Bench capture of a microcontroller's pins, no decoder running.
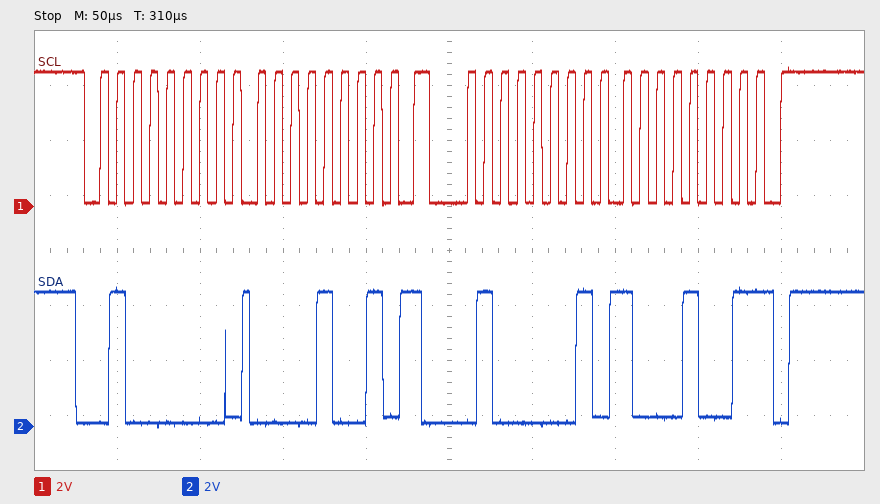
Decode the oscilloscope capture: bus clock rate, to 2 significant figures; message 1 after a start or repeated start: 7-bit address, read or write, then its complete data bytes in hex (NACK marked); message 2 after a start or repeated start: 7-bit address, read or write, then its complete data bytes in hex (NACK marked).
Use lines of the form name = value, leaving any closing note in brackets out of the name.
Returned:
bus clock rate, to 2 significant figures = 100 kHz
message 1 after a start or repeated start: 7-bit address, read or write, then its complete data bytes in hex = 0x20 write: 09
message 2 after a start or repeated start: 7-bit address, read or write, then its complete data bytes in hex = 0x20 read: 89 NACK
